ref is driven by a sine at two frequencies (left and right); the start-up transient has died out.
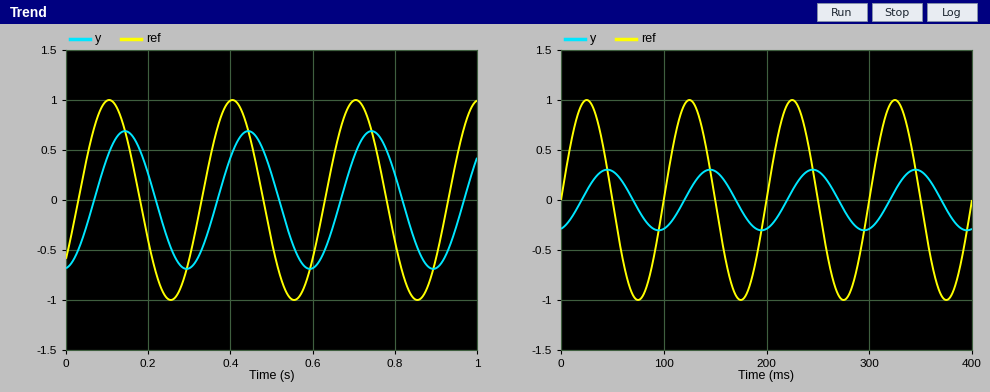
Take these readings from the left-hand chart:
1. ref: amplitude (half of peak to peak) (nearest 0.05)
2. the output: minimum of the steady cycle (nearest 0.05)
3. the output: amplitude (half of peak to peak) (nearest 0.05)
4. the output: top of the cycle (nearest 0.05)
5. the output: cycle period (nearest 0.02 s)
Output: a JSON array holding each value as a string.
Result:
["1.00", "-0.70", "0.70", "0.70", "0.30 s"]
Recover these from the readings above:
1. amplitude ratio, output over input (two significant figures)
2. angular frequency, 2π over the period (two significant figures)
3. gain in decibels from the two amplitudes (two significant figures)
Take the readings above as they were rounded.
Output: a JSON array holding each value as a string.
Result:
["0.70", "21 rad/s", "-3.1 dB"]
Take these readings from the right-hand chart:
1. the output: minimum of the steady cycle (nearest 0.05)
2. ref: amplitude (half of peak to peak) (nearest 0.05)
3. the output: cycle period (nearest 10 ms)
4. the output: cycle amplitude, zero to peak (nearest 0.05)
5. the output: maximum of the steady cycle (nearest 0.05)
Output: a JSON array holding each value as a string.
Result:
["-0.30", "1.00", "100 ms", "0.30", "0.30"]
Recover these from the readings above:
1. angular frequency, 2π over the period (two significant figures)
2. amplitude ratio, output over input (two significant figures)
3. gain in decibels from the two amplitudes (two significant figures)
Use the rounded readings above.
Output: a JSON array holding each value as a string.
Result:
["0.063 rad/ms", "0.30", "-10 dB"]
